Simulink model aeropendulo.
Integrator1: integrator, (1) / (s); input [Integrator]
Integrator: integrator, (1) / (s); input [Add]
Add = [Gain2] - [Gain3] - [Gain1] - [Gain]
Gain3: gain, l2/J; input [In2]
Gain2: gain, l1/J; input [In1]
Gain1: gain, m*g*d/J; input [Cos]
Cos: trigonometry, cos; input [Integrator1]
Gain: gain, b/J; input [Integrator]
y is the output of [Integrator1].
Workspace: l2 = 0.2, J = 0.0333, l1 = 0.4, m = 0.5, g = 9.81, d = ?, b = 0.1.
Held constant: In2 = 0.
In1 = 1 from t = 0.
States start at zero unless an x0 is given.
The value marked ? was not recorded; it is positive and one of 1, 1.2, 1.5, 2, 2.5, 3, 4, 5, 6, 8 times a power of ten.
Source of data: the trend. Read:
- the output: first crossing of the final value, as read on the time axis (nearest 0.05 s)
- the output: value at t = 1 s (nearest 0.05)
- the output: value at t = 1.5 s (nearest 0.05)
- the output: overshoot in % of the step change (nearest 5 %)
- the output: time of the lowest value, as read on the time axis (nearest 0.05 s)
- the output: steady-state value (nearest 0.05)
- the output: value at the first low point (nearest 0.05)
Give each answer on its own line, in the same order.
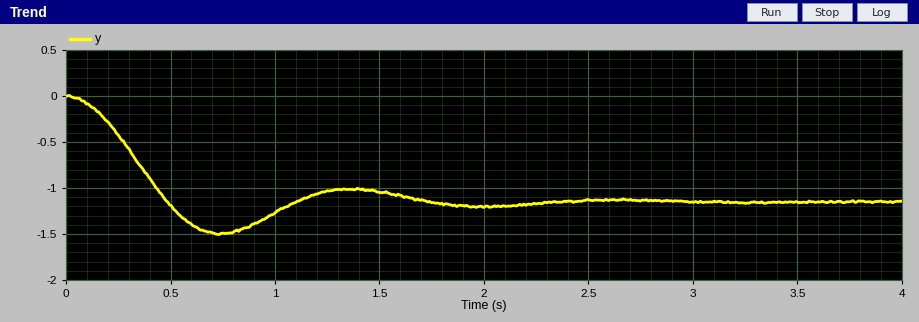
0.50 s
-1.25
-1.05
30 %
0.75 s
-1.15
-1.50
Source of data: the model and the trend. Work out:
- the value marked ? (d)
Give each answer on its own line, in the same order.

0.2
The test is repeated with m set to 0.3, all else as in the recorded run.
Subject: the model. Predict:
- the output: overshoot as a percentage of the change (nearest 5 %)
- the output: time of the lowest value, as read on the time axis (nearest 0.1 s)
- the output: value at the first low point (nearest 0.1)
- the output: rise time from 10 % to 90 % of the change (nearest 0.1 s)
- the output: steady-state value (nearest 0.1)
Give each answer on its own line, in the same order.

15 %
1.2 s
-1.0
0.6 s
-0.8
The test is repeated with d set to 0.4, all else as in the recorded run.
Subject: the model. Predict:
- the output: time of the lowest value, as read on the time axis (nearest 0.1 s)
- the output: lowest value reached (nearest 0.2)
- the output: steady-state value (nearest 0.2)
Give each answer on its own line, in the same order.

0.5 s
-2.0
-1.4
